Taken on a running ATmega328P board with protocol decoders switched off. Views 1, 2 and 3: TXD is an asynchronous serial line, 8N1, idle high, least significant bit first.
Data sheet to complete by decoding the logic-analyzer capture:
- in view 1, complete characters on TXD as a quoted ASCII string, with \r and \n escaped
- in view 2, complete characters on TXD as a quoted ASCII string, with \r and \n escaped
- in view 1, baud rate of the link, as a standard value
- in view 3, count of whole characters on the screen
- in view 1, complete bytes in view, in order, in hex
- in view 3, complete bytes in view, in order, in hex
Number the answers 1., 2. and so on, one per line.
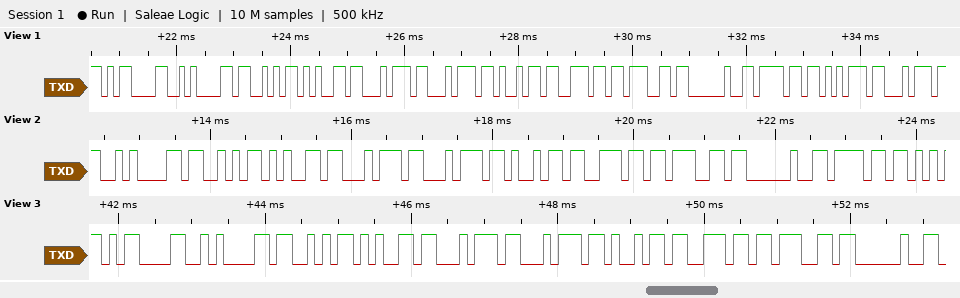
1. "\r\nSetting out"
2. "\nSetting o"
3. 9600 baud
4. 10
5. 0x0D 0x0A 0x53 0x65 0x74 0x74 0x69 0x6E 0x67 0x20 0x6F 0x75 0x74
6. 0D 0A 53 65 74 74 69 6E 67 20
